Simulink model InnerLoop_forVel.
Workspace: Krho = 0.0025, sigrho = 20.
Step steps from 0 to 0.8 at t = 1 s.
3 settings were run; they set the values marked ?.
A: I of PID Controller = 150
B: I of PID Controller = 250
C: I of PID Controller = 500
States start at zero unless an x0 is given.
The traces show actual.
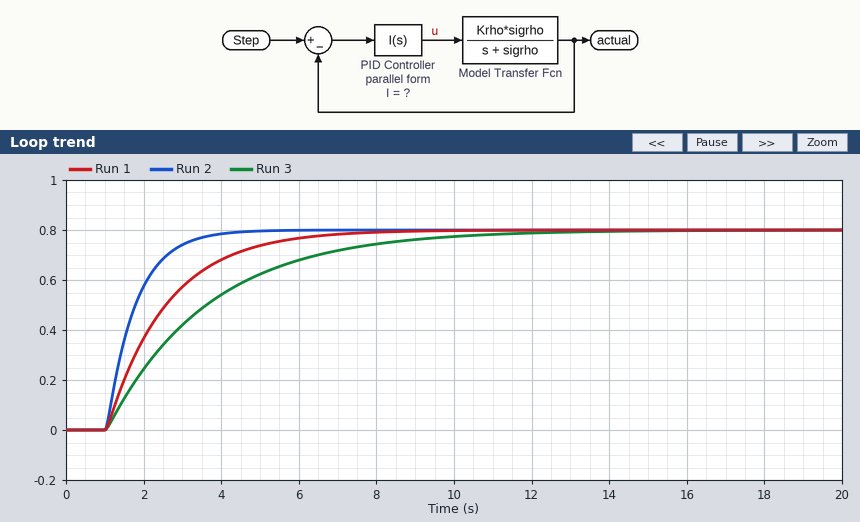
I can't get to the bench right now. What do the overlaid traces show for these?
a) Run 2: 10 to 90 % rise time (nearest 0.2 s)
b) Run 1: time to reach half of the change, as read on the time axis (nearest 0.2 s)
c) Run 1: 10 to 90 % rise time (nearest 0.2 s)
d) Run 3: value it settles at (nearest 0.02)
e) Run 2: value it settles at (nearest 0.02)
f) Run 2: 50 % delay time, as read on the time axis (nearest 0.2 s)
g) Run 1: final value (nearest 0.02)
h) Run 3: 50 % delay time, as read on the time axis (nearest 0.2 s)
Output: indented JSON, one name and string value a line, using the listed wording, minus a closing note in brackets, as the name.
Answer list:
{
  "Run 2: 10 to 90 % rise time": "1.6 s",
  "Run 1: time to reach half of the change, as read on the time axis": "2.2 s",
  "Run 1: 10 to 90 % rise time": "3.4 s",
  "Run 3: value it settles at": "0.80",
  "Run 2: value it settles at": "0.80",
  "Run 2: 50 % delay time, as read on the time axis": "1.6 s",
  "Run 1: final value": "0.80",
  "Run 3: 50 % delay time, as read on the time axis": "2.8 s"
}
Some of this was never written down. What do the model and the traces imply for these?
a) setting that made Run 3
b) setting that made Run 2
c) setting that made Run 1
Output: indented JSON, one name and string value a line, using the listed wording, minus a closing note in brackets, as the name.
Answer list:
{
  "setting that made Run 3": "A",
  "setting that made Run 2": "C",
  "setting that made Run 1": "B"
}
